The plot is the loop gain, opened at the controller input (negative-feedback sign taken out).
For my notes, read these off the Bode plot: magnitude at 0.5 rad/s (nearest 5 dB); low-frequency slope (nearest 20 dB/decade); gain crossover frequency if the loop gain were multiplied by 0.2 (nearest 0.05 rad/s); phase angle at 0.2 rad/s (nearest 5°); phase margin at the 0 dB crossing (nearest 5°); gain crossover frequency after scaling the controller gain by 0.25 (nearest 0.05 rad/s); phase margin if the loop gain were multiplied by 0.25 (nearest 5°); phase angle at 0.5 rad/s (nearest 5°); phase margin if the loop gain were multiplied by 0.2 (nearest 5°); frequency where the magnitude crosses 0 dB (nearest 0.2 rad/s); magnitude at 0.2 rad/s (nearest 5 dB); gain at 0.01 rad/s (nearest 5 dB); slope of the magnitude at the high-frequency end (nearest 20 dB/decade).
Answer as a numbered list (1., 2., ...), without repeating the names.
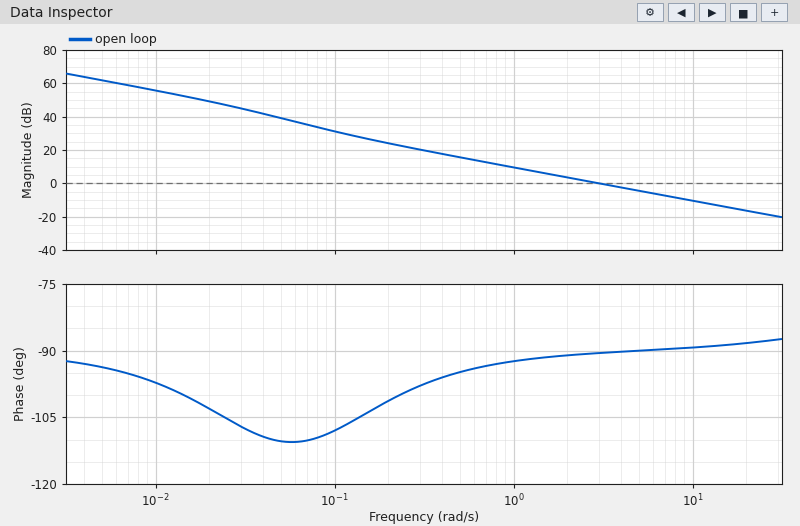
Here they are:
1. 15 dB
2. -20 dB/decade
3. 0.60 rad/s
4. -100°
5. 90°
6. 0.75 rad/s
7. 85°
8. -95°
9. 85°
10. 3.0 rad/s
11. 25 dB
12. 55 dB
13. -20 dB/decade
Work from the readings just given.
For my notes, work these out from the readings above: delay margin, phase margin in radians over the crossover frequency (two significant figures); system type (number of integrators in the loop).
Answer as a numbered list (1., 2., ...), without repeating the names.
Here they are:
1. 0.52 s
2. 1
